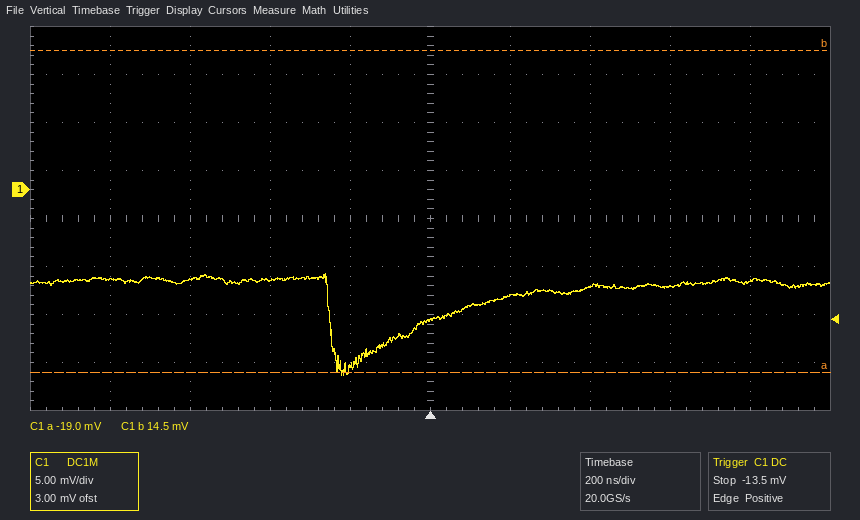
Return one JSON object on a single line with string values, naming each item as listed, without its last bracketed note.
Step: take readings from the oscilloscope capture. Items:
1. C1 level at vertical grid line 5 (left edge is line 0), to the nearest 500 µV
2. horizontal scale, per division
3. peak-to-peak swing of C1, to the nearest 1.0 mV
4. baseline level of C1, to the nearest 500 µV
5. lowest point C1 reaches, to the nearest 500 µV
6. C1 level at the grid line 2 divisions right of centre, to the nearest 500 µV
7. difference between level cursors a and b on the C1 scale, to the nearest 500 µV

{"C1 level at vertical grid line 5 (left edge is line 0), to the nearest 500 µV": "-13.5 mV", "horizontal scale, per division": "200 ns", "peak-to-peak swing of C1, to the nearest 1.0 mV": "11.0 mV", "baseline level of C1, to the nearest 500 µV": "-9.5 mV", "lowest point C1 reaches, to the nearest 500 µV": "-19.5 mV", "C1 level at the grid line 2 divisions right of centre, to the nearest 500 µV": "-10.0 mV", "difference between level cursors a and b on the C1 scale, to the nearest 500 µV": "33.5 mV"}
